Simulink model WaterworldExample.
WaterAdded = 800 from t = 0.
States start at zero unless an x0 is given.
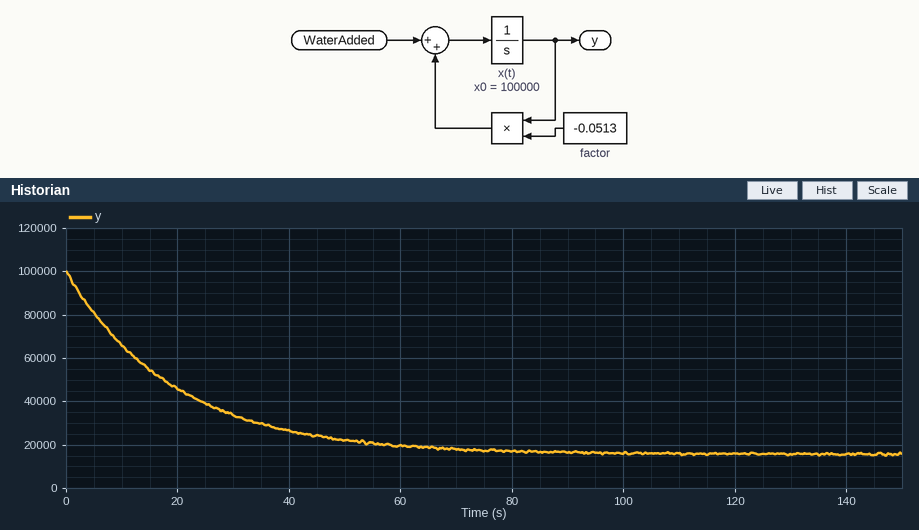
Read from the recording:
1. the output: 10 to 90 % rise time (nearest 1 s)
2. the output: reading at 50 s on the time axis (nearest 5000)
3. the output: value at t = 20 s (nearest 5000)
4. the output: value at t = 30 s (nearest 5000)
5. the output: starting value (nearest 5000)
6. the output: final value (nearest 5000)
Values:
43 s
20000
45000
35000
100000
15000
